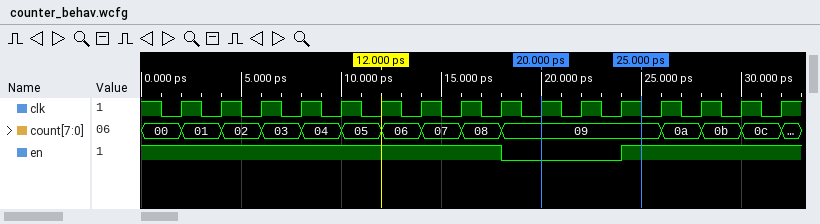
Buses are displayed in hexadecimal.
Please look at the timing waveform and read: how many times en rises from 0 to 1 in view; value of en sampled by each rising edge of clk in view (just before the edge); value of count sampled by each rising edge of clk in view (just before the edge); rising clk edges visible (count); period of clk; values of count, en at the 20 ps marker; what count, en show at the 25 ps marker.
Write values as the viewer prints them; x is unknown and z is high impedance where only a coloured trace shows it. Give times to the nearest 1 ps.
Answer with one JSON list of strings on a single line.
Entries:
["1", "1 1 1 1 1 1 1 1 1 0 0 0 1 1 1 1", "00, 01, 02, 03, 04, 05, 06, 07, 08, 09, 09, 09, 09, 0a, 0b, 0c", "16", "2 ps", "count=09, en=0", "count=09, en=1"]
